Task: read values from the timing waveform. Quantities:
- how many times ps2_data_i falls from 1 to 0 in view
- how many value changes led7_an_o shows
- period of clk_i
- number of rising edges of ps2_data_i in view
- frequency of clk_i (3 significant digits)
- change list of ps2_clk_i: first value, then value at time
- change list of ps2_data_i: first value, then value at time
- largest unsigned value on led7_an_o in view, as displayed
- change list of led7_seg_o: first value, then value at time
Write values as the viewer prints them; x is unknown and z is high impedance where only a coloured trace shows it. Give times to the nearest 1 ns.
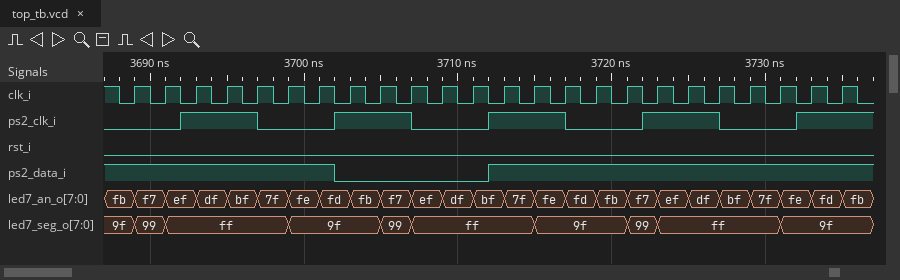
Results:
1
24
2 ns
1
500 MHz
0, 1 at 3692 ns, 0 at 3697 ns, 1 at 3702 ns, 0 at 3707 ns, 1 at 3712 ns, 0 at 3717 ns, 1 at 3722 ns, 0 at 3727 ns, 1 at 3732 ns
1, 0 at 3702 ns, 1 at 3712 ns
fe
9f, 99 at 3689 ns, ff at 3691 ns, 9f at 3699 ns, 99 at 3705 ns, ff at 3707 ns, 9f at 3715 ns, 99 at 3721 ns, ff at 3723 ns, 9f at 3731 ns
